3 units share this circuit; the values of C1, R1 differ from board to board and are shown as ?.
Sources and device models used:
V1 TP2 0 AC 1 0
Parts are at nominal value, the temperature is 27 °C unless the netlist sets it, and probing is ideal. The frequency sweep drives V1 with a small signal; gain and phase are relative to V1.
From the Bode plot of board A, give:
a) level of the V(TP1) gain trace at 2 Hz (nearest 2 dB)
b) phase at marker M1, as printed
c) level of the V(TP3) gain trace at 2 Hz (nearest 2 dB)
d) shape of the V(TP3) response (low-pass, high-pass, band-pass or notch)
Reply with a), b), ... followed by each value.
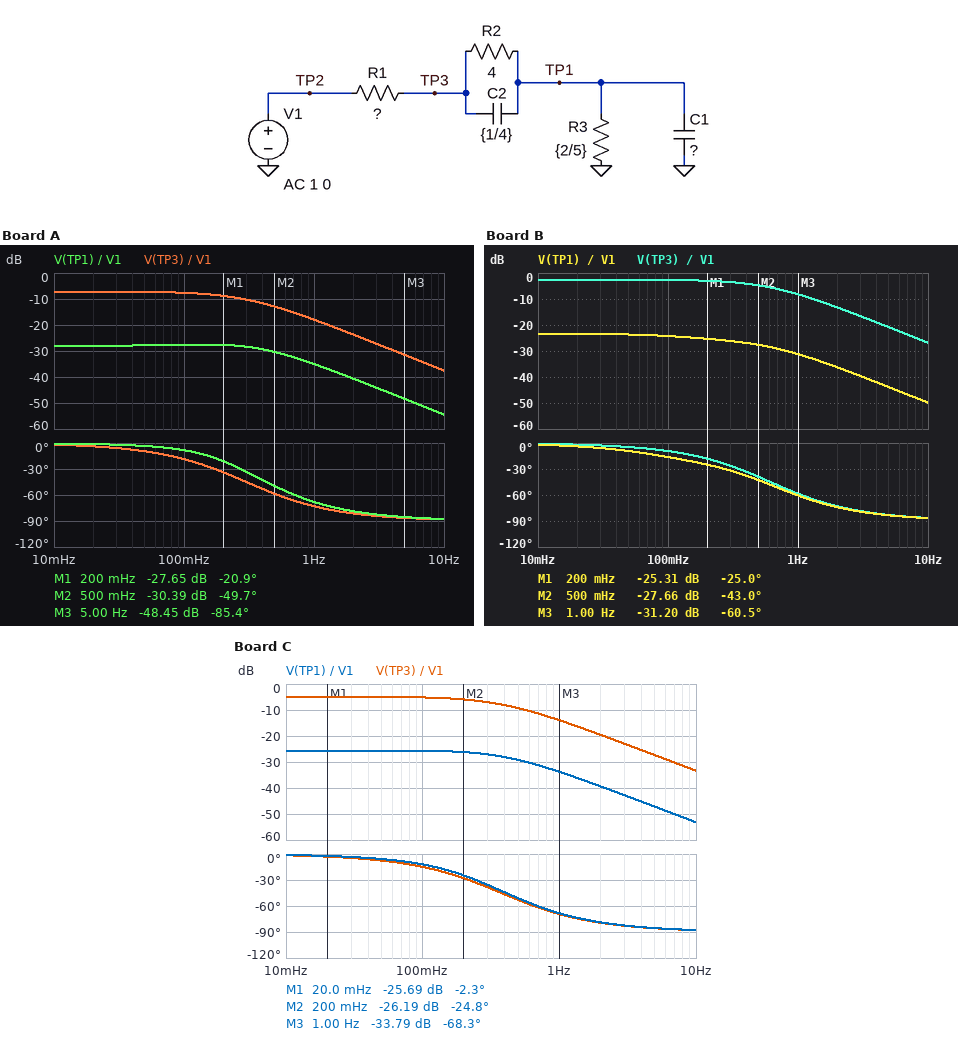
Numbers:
a) -40 dB
b) -20.9 deg
c) -24 dB
d) low-pass
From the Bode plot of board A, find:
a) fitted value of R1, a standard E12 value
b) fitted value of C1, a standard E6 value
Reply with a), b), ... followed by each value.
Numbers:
a) 5.6 Ω
b) 1.5 F
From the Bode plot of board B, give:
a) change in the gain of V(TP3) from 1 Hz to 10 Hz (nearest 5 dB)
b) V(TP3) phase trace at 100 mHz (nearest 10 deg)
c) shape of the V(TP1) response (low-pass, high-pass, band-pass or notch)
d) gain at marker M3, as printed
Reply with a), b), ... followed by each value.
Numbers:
a) -20 dB
b) -10 deg
c) low-pass
d) -31.20 dB
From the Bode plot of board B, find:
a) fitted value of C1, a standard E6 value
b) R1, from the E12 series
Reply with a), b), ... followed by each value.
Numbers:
a) 3.3 F
b) 1.5 Ω
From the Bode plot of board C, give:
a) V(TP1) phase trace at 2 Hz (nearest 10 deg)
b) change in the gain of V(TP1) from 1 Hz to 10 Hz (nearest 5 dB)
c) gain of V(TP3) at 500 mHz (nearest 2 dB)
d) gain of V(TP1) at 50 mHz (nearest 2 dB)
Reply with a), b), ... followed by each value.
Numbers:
a) -80 deg
b) -20 dB
c) -10 dB
d) -26 dB
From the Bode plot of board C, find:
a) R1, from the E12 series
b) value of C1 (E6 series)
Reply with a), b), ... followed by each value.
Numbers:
a) 3.3 Ω
b) 2.2 F
